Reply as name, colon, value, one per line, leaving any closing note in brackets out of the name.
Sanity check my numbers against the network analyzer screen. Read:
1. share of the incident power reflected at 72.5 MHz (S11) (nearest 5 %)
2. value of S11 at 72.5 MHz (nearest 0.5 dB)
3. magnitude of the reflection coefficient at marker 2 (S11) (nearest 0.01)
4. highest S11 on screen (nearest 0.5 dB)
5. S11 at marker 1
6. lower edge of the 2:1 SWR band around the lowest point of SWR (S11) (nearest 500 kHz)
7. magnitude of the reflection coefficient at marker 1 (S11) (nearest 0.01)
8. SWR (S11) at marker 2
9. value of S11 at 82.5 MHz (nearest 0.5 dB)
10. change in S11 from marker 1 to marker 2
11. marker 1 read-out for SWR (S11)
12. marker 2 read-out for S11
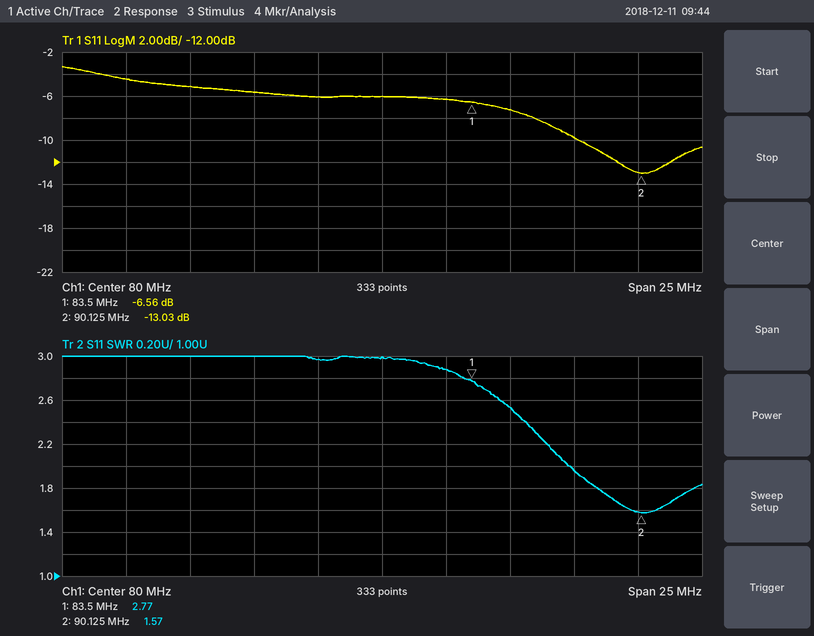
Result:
share of the incident power reflected at 72.5 MHz (S11): 30 %
value of S11 at 72.5 MHz: -5.0 dB
magnitude of the reflection coefficient at marker 2 (S11): 0.22
highest S11 on screen: -3.5 dB
S11 at marker 1: -6.56 dB
lower edge of the 2:1 SWR band around the lowest point of SWR (S11): 87.5 MHz
magnitude of the reflection coefficient at marker 1 (S11): 0.47
SWR (S11) at marker 2: 1.57
value of S11 at 82.5 MHz: -6.5 dB
change in S11 from marker 1 to marker 2: -6.47 dB
marker 1 read-out for SWR: 2.77
marker 2 read-out for S11: -13.03 dB
